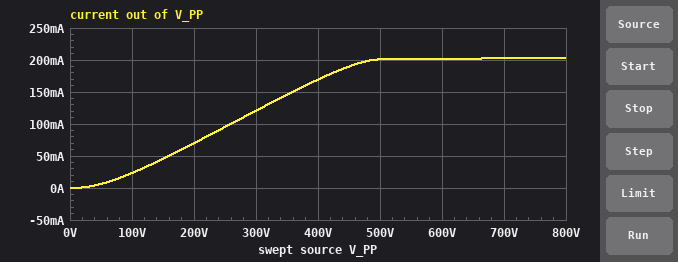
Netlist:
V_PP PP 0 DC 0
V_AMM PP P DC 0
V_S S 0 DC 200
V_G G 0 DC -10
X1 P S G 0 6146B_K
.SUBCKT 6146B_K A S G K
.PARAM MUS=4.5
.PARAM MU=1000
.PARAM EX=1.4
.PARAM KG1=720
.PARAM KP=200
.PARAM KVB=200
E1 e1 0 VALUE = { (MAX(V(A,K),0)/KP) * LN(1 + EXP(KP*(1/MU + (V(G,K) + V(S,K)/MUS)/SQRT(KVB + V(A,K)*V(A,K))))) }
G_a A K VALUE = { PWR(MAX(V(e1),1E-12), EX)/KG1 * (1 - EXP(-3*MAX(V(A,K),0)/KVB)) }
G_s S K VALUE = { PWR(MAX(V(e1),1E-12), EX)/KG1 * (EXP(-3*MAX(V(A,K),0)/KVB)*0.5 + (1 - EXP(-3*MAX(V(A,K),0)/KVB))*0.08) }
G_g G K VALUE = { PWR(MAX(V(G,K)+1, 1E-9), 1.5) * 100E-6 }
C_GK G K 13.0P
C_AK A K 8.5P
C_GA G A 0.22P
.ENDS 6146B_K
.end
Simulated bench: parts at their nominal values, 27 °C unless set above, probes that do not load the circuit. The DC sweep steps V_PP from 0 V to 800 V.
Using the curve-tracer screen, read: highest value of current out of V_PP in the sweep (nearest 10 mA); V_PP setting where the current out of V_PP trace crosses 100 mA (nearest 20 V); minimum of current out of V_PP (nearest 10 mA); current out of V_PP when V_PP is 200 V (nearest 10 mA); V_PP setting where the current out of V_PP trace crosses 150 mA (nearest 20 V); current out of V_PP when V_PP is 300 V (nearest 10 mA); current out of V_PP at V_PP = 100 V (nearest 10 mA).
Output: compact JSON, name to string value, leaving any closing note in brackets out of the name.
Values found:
{"highest value of current out of V_PP in the sweep": "200 mA", "V_PP setting where the current out of V_PP trace crosses 100 mA": "260 V", "minimum of current out of V_PP": "0 A", "current out of V_PP when V_PP is 200 V": "70 mA", "V_PP setting where the current out of V_PP trace crosses 150 mA": "360 V", "current out of V_PP when V_PP is 300 V": "120 mA", "current out of V_PP at V_PP = 100 V": "20 mA"}
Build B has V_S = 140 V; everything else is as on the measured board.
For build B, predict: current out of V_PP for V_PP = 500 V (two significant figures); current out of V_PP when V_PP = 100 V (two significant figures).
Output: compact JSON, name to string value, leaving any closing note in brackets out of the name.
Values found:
{"current out of V_PP for V_PP = 500 V": "100 mA", "current out of V_PP when V_PP = 100 V": "22 mA"}
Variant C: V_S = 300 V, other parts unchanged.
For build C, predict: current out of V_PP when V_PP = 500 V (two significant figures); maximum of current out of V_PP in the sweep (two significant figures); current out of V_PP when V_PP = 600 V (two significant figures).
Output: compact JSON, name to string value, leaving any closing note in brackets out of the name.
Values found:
{"current out of V_PP when V_PP = 500 V": "250 mA", "maximum of current out of V_PP in the sweep": "400 mA", "current out of V_PP when V_PP = 600 V": "310 mA"}
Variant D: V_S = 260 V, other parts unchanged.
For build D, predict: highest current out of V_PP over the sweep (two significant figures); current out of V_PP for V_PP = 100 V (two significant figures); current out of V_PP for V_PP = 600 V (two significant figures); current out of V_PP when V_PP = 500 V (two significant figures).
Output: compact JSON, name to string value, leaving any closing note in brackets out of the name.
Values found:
{"highest current out of V_PP over the sweep": "320 mA", "current out of V_PP for V_PP = 100 V": "24 mA", "current out of V_PP for V_PP = 600 V": "290 mA", "current out of V_PP when V_PP = 500 V": "240 mA"}
